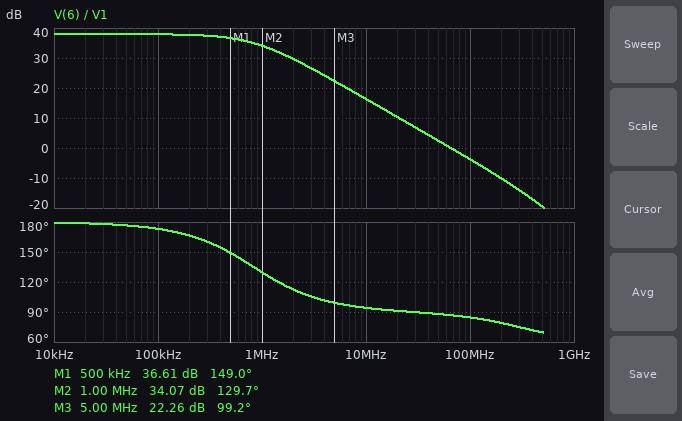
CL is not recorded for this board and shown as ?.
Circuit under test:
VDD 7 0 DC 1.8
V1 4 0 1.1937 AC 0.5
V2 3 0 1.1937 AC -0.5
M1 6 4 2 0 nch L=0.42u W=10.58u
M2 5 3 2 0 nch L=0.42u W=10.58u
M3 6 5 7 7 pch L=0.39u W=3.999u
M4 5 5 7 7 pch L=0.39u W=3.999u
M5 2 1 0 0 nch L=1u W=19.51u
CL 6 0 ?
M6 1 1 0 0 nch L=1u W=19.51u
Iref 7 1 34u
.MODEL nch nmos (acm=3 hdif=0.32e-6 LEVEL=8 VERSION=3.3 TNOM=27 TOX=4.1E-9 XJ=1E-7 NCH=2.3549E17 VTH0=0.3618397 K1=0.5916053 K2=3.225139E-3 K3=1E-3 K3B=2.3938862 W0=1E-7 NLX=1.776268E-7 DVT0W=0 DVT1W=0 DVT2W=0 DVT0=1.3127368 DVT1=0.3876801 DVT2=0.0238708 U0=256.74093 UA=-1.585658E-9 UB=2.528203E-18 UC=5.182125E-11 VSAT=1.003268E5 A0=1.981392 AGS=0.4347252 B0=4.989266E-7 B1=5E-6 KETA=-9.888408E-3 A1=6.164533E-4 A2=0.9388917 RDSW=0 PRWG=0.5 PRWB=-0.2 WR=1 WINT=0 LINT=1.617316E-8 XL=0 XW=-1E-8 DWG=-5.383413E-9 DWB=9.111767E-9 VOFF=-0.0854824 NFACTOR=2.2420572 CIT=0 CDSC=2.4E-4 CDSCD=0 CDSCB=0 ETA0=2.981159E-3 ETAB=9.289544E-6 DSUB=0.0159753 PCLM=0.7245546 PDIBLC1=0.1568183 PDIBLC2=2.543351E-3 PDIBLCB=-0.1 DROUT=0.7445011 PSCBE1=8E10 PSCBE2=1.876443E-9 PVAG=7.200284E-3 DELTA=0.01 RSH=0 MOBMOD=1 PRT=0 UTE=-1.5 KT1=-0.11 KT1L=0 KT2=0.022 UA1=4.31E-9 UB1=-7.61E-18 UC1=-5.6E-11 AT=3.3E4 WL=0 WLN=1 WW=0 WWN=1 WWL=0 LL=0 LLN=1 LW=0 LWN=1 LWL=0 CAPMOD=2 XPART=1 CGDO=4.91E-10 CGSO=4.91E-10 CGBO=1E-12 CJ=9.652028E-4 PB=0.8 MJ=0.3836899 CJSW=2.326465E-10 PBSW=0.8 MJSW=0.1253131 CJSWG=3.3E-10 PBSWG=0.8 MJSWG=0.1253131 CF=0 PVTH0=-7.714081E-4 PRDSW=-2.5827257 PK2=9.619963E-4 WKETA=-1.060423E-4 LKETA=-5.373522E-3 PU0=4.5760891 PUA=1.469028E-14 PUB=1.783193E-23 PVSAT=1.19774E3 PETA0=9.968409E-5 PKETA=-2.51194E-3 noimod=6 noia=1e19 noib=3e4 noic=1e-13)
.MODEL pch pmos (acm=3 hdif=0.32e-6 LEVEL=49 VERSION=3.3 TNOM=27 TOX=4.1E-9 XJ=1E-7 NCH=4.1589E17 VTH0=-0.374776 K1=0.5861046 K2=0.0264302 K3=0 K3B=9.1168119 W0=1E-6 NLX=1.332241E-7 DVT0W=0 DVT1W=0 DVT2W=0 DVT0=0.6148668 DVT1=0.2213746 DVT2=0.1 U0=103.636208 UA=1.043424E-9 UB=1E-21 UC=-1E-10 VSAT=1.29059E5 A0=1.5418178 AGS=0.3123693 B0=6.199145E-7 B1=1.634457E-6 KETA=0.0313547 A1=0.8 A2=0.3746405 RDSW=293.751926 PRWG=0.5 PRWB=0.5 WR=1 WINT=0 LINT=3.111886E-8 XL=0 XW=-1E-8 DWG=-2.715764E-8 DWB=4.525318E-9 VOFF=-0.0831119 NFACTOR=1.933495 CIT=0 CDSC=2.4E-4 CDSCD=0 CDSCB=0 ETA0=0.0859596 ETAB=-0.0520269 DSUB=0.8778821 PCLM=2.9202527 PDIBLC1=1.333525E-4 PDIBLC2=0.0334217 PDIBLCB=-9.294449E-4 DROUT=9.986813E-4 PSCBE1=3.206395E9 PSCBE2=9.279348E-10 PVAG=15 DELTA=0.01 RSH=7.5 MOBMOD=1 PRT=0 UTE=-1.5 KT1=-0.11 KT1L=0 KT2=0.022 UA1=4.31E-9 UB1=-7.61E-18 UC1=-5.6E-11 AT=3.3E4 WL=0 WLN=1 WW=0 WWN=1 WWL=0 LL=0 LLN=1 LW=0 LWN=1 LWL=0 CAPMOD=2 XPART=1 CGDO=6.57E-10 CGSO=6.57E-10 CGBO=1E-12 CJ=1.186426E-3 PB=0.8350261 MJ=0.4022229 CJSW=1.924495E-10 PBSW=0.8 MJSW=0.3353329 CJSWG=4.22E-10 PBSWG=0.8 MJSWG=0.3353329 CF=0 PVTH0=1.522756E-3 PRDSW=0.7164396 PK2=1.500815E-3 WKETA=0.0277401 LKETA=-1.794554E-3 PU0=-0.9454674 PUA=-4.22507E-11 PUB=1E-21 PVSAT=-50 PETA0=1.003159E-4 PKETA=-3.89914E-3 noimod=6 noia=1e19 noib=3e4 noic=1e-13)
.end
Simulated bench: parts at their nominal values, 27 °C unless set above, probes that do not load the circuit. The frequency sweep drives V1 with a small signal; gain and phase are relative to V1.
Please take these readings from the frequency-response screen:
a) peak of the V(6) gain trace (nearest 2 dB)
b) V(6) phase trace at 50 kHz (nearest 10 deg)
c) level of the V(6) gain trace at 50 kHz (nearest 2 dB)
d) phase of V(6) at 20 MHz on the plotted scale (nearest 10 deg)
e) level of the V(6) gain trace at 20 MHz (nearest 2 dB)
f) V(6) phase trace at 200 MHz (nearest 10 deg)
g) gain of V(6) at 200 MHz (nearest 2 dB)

38 dB
180 deg
38 dB
90 deg
10 dB
80 deg
-10 dB
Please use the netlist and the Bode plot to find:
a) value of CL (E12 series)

1.2 pF
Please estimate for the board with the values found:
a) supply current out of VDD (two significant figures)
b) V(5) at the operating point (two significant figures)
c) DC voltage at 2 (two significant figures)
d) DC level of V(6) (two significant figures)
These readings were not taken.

68 µA
1.1 V
540 mV
1.1 V
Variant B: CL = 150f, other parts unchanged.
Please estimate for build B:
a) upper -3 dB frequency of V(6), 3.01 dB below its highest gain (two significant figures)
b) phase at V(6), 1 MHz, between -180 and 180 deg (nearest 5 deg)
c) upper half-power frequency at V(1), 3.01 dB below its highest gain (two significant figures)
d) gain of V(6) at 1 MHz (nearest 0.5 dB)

5.8 MHz
170 deg
3.8 GHz
38.0 dB
